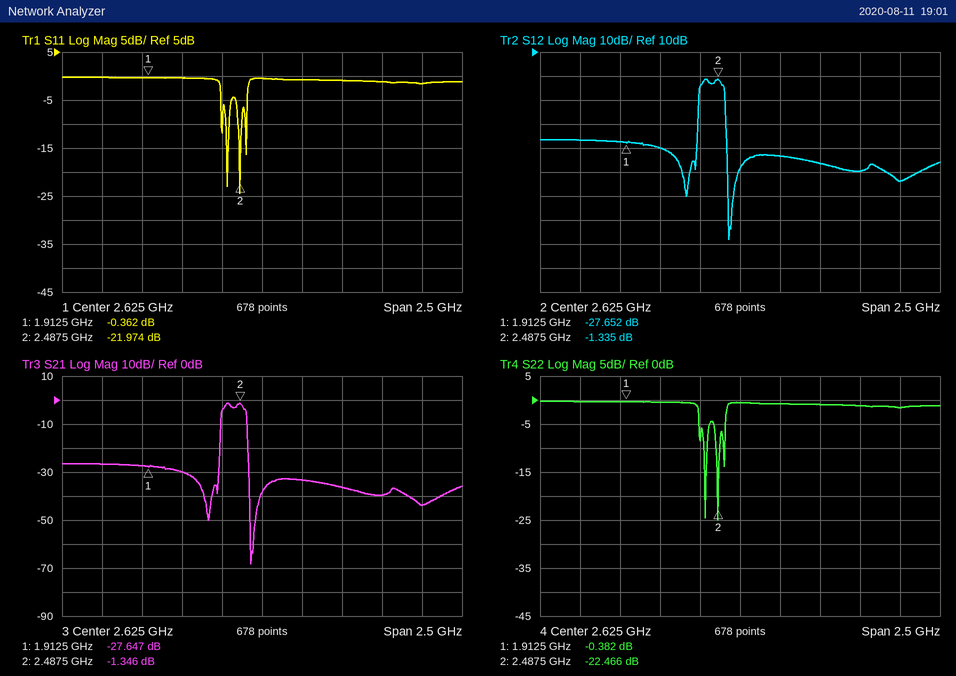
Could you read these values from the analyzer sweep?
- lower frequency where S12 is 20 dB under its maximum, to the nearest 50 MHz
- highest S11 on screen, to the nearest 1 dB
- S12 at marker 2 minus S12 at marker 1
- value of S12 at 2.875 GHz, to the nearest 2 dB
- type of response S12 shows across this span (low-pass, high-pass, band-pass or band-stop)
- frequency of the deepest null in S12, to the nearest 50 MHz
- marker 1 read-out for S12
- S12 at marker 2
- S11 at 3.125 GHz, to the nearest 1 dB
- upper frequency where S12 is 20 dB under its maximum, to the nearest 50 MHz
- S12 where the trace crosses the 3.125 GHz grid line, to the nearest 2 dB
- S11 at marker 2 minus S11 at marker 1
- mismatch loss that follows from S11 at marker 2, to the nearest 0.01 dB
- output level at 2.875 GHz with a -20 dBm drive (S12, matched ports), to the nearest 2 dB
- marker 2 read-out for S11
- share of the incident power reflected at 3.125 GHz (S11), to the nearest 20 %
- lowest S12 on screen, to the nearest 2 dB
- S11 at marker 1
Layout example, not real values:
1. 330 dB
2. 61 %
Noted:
1. 2.35 GHz
2. 0 dB
3. 26.317 dB
4. -34 dB
5. band-pass
6. 2.55 GHz
7. -27.652 dB
8. -1.335 dB
9. -1 dB
10. 2.55 GHz
11. -36 dB
12. -21.612 dB
13. 0.03 dB
14. -54 dBm
15. -21.974 dB
16. 80 %
17. -68 dB
18. -0.362 dB
